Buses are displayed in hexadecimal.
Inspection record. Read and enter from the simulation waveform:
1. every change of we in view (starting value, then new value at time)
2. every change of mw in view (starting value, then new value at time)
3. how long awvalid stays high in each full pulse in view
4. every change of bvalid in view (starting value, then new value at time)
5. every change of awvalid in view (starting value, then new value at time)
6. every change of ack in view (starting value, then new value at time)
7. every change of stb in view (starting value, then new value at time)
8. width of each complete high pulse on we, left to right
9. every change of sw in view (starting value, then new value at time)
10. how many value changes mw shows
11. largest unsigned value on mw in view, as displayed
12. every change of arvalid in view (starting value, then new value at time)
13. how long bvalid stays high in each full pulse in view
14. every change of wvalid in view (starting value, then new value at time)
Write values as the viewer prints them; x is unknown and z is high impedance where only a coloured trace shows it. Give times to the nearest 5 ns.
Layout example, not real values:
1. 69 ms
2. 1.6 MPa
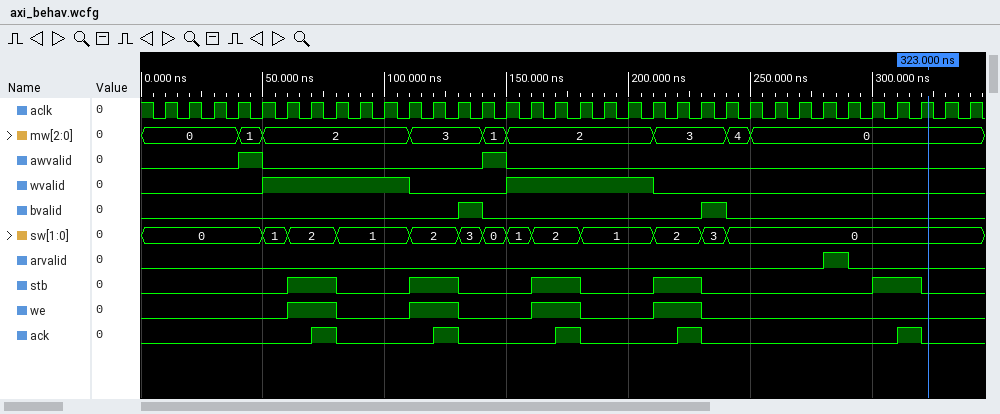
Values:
1. 0, 1 at 60 ns, 0 at 80 ns, 1 at 110 ns, 0 at 130 ns, 1 at 160 ns, 0 at 180 ns, 1 at 210 ns, 0 at 230 ns
2. 0, 1 at 40 ns, 2 at 50 ns, 3 at 110 ns, 1 at 140 ns, 2 at 150 ns, 3 at 210 ns, 4 at 240 ns, 0 at 250 ns
3. 10 ns, 10 ns
4. 0, 1 at 130 ns, 0 at 140 ns, 1 at 230 ns, 0 at 240 ns
5. 0, 1 at 40 ns, 0 at 50 ns, 1 at 140 ns, 0 at 150 ns
6. 0, 1 at 70 ns, 0 at 80 ns, 1 at 120 ns, 0 at 130 ns, 1 at 170 ns, 0 at 180 ns, 1 at 220 ns, 0 at 230 ns, 1 at 310 ns, 0 at 320 ns
7. 0, 1 at 60 ns, 0 at 80 ns, 1 at 110 ns, 0 at 130 ns, 1 at 160 ns, 0 at 180 ns, 1 at 210 ns, 0 at 230 ns, 1 at 300 ns, 0 at 320 ns
8. 20 ns, 20 ns, 20 ns, 20 ns
9. 0, 1 at 50 ns, 2 at 60 ns, 1 at 80 ns, 2 at 110 ns, 3 at 130 ns, 0 at 140 ns, 1 at 150 ns, 2 at 160 ns, 1 at 180 ns, 2 at 210 ns, 3 at 230 ns, 0 at 240 ns
10. 8
11. 4
12. 0, 1 at 280 ns, 0 at 290 ns
13. 10 ns, 10 ns
14. 0, 1 at 50 ns, 0 at 110 ns, 1 at 150 ns, 0 at 210 ns
